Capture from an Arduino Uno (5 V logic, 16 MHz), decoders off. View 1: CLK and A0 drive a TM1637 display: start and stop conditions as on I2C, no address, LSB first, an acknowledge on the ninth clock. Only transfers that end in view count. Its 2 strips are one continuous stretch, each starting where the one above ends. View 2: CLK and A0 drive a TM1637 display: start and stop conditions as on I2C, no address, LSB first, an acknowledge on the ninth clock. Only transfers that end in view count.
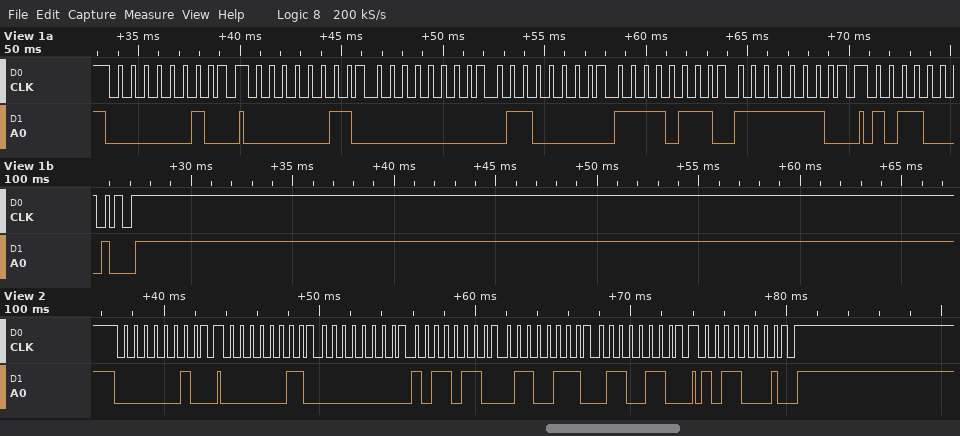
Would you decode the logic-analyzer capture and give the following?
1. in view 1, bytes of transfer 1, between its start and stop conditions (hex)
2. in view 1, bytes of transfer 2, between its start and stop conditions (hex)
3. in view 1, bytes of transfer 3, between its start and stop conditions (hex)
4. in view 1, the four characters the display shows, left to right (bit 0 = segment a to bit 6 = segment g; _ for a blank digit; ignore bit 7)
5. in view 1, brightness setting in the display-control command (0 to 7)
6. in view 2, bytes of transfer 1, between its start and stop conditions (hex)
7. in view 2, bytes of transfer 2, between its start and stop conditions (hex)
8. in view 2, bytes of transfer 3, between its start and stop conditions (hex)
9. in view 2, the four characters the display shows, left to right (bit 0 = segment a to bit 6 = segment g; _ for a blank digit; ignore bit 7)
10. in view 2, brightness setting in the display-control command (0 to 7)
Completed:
40
C0 00 06 EF 7F
8D
_198
5
40
C0 00 6D E6 66
8D
_544
5
